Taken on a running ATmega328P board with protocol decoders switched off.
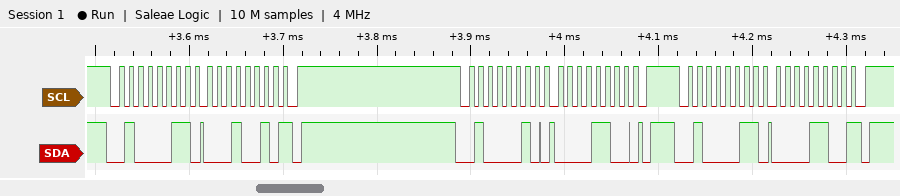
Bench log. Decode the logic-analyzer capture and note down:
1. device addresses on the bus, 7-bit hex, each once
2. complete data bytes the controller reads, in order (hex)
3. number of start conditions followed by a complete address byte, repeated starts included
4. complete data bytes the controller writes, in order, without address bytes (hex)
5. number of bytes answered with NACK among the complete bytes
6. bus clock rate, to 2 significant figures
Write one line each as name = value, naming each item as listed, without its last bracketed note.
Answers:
device addresses on the bus, 7-bit hex, each once = 0x21
complete data bytes the controller reads, in order = 12 0C
number of start conditions followed by a complete address byte, repeated starts included = 3
complete data bytes the controller writes, in order, without address bytes = 0C
number of bytes answered with NACK among the complete bytes = 2
bus clock rate, to 2 significant figures = 100 kHz
